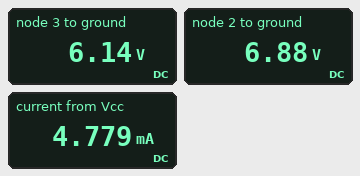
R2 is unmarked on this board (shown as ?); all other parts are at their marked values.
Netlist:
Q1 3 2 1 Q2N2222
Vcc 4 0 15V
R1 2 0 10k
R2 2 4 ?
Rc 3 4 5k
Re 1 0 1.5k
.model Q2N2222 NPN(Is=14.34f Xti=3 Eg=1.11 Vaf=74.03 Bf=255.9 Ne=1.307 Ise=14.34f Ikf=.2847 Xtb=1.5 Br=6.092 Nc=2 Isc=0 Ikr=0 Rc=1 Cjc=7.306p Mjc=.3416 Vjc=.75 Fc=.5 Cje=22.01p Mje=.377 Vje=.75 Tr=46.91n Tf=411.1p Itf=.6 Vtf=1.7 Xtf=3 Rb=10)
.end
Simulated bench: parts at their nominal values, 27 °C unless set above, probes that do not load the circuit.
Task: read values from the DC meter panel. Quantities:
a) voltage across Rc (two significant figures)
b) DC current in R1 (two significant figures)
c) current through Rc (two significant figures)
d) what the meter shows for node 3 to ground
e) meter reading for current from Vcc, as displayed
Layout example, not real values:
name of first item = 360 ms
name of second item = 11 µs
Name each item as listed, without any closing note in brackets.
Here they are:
voltage across Rc = 8.9 V
DC current in R1 = 690 µA
current through Rc = 1.8 mA
what the meter shows for node 3 to ground = 6.14 V
meter reading for current from Vcc, as displayed = 4.779 mA
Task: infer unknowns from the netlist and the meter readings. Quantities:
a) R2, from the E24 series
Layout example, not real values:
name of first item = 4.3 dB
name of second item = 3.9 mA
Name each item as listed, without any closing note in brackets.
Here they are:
R2, from the E24 series = 2.7 kΩ
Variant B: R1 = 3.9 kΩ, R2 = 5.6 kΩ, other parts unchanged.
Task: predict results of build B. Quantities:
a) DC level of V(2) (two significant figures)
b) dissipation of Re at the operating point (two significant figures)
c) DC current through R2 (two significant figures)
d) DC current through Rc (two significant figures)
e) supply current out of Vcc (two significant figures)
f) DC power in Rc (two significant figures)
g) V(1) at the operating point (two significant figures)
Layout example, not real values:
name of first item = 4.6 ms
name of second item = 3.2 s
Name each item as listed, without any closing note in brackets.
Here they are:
DC level of V(2) = 4.8 V
dissipation of Re at the operating point = 11 mW
DC current through R2 = 1.8 mA
DC current through Rc = 2.2 mA
supply current out of Vcc = 4.0 mA
DC power in Rc = 24 mW
V(1) at the operating point = 4.1 V
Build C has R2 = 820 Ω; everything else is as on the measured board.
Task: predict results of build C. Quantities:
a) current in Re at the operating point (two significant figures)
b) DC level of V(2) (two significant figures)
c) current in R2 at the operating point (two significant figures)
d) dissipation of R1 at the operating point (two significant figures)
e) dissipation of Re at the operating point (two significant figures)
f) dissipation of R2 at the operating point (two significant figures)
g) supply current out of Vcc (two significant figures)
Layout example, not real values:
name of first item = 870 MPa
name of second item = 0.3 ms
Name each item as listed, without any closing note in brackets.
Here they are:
current in Re at the operating point = 6.2 mA
DC level of V(2) = 10 V
current in R2 at the operating point = 6.0 mA
dissipation of R1 at the operating point = 10 mW
dissipation of Re at the operating point = 57 mW
dissipation of R2 at the operating point = 30 mW
supply current out of Vcc = 7.2 mA
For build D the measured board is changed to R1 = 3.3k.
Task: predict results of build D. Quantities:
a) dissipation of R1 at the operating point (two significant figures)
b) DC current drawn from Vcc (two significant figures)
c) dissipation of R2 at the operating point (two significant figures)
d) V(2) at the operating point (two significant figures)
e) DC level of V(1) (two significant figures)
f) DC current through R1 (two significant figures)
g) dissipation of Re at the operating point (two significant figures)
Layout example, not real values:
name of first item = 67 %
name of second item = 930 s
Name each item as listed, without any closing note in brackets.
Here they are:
dissipation of R1 at the operating point = 11 mW
DC current drawn from Vcc = 5.3 mA
dissipation of R2 at the operating point = 30 mW
V(2) at the operating point = 6.0 V
DC level of V(1) = 5.2 V
DC current through R1 = 1.8 mA
dissipation of Re at the operating point = 18 mW
